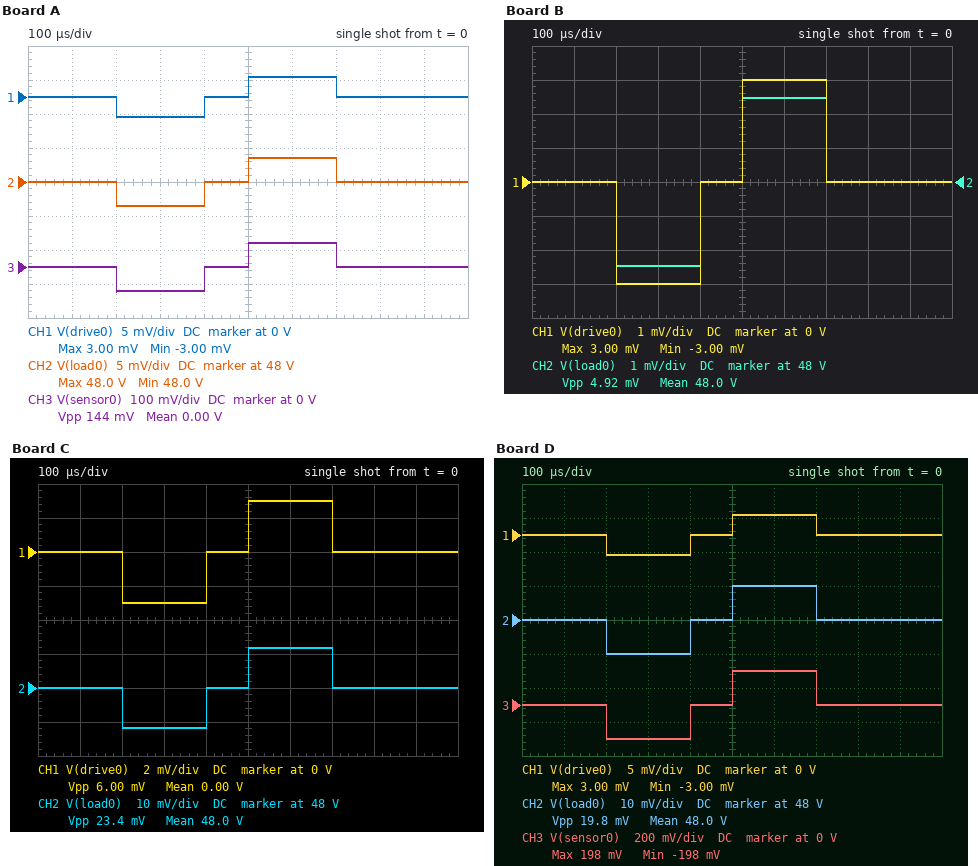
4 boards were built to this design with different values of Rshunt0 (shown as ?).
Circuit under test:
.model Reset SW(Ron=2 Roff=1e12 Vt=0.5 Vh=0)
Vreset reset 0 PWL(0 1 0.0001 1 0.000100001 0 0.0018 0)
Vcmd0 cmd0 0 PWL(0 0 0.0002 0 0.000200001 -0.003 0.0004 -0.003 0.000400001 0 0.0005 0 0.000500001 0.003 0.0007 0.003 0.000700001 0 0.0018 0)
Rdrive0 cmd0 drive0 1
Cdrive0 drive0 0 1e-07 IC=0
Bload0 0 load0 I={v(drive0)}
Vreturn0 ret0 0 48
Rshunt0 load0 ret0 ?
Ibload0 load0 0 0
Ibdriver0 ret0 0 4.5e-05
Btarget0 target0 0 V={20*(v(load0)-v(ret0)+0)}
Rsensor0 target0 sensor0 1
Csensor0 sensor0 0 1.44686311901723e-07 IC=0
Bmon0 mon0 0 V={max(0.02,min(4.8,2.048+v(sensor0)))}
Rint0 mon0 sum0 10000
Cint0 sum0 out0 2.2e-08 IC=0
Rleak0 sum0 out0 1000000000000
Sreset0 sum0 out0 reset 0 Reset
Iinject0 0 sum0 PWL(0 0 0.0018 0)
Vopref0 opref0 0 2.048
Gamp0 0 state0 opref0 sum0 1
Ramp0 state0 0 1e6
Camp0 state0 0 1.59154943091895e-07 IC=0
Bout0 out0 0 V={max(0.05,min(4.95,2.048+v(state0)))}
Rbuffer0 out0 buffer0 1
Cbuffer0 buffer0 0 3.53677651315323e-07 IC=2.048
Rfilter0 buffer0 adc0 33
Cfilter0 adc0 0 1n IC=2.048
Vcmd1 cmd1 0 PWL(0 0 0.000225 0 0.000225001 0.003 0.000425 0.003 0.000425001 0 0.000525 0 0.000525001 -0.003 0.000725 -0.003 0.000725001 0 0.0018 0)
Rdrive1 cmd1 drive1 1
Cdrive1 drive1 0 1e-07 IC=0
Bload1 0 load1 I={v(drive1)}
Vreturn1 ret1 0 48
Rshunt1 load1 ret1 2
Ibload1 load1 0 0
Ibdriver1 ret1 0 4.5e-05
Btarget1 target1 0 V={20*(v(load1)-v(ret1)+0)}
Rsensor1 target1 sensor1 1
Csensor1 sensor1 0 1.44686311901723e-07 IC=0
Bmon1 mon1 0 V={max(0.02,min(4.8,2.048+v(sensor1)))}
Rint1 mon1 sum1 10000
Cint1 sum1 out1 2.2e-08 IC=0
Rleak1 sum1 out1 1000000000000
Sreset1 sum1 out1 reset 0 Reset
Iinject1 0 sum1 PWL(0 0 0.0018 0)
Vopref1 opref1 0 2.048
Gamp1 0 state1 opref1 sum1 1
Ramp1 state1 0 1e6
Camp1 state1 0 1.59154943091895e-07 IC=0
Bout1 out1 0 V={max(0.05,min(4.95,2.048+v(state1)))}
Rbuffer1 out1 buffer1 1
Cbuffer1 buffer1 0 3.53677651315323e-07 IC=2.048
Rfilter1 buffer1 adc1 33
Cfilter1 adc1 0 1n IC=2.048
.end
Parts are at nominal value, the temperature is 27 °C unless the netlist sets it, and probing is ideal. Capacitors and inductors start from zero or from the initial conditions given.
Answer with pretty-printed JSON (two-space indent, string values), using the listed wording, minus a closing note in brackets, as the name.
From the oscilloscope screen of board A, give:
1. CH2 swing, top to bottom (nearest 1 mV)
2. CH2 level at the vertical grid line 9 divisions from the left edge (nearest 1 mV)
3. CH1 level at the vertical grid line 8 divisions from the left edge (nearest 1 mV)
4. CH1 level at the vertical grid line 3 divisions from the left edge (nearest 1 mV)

{
  "CH2 swing, top to bottom": "7 mV",
  "CH2 level at the vertical grid line 9 divisions from the left edge": "48.000 V",
  "CH1 level at the vertical grid line 8 divisions from the left edge": "0 V",
  "CH1 level at the vertical grid line 3 divisions from the left edge": "-3 mV"
}
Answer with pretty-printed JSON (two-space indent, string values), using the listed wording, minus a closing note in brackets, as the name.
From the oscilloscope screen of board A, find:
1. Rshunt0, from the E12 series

{
  "Rshunt0, from the E12 series": "1.2 Ω"
}
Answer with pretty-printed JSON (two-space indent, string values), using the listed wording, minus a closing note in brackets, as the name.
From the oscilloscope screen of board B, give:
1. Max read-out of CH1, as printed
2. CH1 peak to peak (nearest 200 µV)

{
  "Max read-out of CH1, as printed": "3.00 mV",
  "CH1 peak to peak": "6.0 mV"
}
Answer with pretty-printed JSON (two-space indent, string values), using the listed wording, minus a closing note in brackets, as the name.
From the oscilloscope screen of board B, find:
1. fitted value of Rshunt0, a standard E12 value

{
  "fitted value of Rshunt0, a standard E12 value": "0.82 Ω"
}
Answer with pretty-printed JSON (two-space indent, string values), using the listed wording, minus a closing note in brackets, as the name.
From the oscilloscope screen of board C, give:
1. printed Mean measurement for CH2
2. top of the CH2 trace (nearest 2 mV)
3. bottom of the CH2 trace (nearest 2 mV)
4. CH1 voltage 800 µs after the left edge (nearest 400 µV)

{
  "printed Mean measurement for CH2": "48.0 V",
  "top of the CH2 trace": "48.012 V",
  "bottom of the CH2 trace": "47.988 V",
  "CH1 voltage 800 µs after the left edge": "0 V"
}
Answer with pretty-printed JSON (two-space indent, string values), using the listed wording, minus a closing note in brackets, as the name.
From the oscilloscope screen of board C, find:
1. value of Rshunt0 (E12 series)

{
  "value of Rshunt0": "3.9 Ω"
}
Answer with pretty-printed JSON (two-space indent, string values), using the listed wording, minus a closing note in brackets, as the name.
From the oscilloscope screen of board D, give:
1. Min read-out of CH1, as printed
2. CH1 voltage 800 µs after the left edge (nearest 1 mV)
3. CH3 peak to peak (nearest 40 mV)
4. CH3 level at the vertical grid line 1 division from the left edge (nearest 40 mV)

{
  "Min read-out of CH1, as printed": "-3.00 mV",
  "CH1 voltage 800 µs after the left edge": "0 V",
  "CH3 peak to peak": "400 mV",
  "CH3 level at the vertical grid line 1 division from the left edge": "0 V"
}
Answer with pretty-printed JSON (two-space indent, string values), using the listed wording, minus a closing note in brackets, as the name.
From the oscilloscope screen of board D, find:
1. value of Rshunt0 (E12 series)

{
  "value of Rshunt0": "3.3 Ω"
}
